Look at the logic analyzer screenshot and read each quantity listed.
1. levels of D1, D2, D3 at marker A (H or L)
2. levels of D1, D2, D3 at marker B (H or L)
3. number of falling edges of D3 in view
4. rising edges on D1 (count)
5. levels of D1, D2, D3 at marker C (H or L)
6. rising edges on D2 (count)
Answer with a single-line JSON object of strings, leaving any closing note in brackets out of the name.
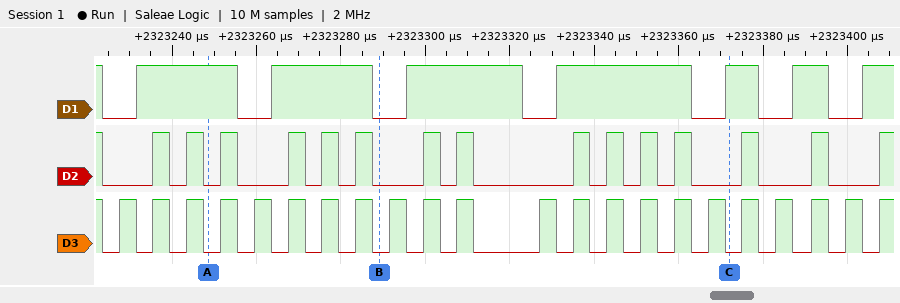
{"levels of D1, D2, D3 at marker A": "D1=H, D2=L, D3=L", "levels of D1, D2, D3 at marker B": "D1=L, D2=L, D3=L", "number of falling edges of D3 in view": "22", "rising edges on D1": "7", "levels of D1, D2, D3 at marker C": "D1=H, D2=L, D3=L", "rising edges on D2": "15"}
